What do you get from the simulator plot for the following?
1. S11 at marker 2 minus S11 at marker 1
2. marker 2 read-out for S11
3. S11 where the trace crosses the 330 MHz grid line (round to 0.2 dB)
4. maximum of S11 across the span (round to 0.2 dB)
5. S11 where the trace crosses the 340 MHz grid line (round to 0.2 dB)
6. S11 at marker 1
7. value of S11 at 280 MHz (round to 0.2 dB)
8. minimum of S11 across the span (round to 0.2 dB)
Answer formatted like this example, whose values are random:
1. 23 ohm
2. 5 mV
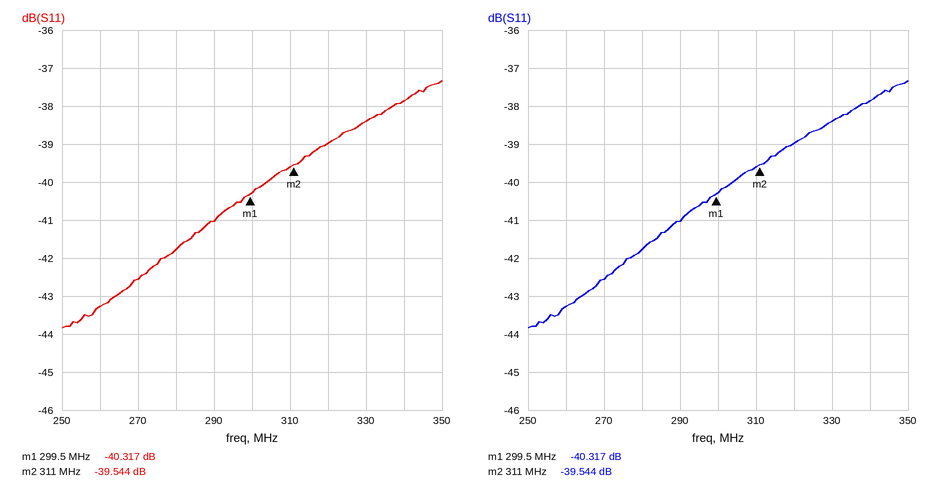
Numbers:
1. 0.773 dB
2. -39.544 dB
3. -38.4 dB
4. -37.4 dB
5. -37.8 dB
6. -40.317 dB
7. -41.8 dB
8. -43.8 dB
